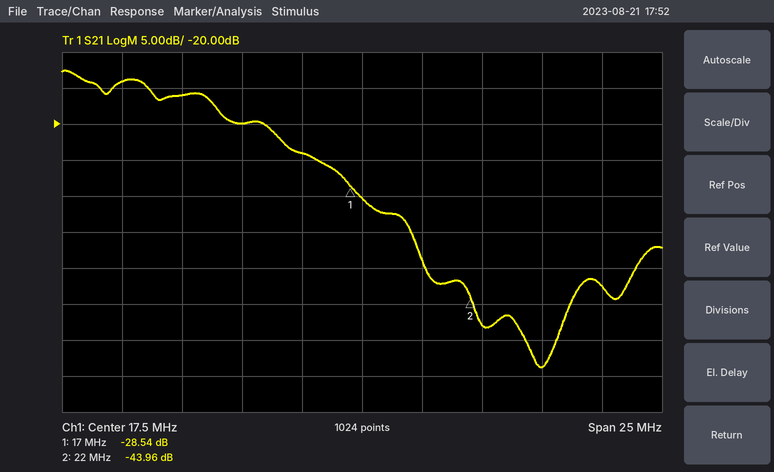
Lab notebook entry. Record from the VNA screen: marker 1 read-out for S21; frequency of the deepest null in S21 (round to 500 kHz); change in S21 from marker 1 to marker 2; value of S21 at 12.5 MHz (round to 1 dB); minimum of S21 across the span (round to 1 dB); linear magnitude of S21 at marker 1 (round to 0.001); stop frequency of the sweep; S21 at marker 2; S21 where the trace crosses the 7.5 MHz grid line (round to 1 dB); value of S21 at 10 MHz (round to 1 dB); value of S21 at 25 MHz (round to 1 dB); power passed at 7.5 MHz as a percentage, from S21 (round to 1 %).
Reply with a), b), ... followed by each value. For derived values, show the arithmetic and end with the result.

a) -28.54 dB
b) 25.0 MHz
c) -43.96 − (-28.54) = -15.42 dB
d) -20 dB
e) -54 dB
f) 10^(-28.54/20) ≈ 0.037
g) 30 MHz
h) -43.96 dB
i) -14 dB
j) -16 dB
k) -54 dB
l) 10^(-14/10) ≈ 4 %
